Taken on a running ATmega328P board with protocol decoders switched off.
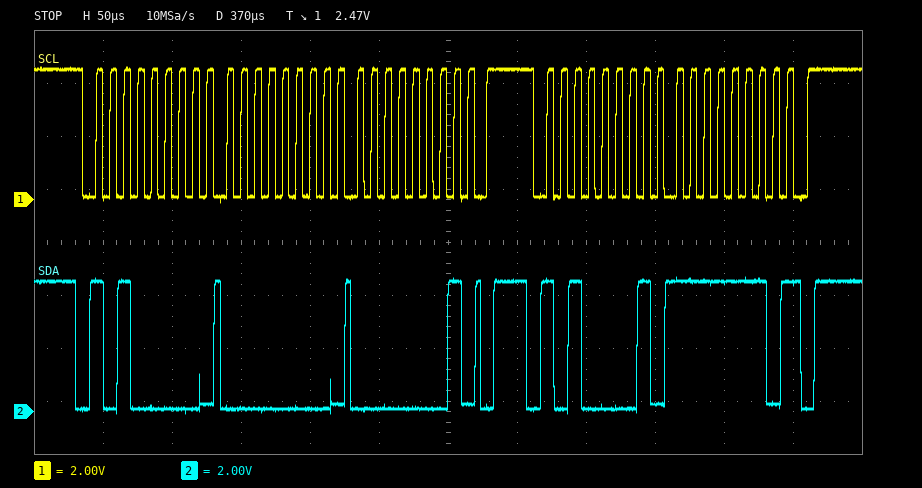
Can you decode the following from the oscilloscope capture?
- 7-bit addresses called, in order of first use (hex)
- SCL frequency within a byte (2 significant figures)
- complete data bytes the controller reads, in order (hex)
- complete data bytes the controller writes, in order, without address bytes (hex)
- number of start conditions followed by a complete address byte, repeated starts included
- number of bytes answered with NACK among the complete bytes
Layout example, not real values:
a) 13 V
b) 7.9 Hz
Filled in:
a) 0x50
b) 100 kHz
c) FE
d) 00 01
e) 2
f) 1
